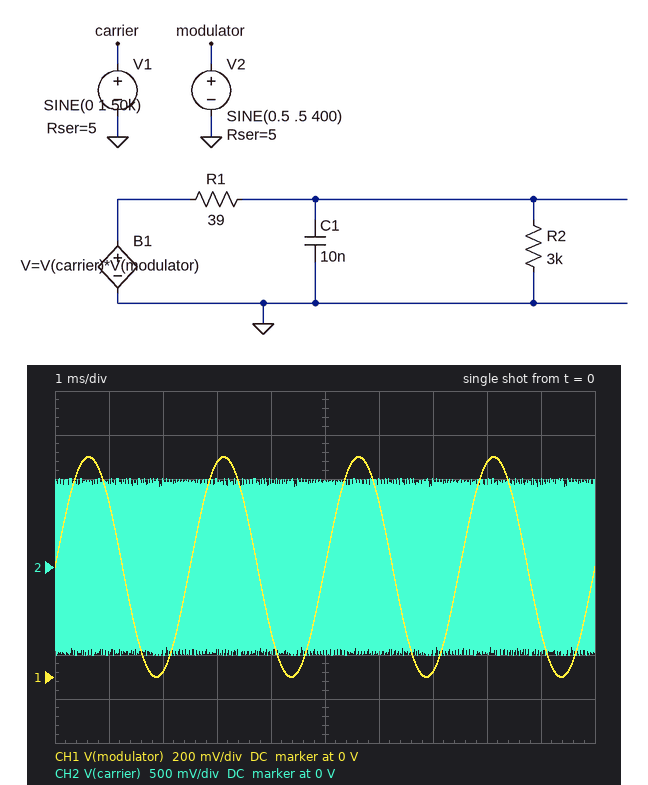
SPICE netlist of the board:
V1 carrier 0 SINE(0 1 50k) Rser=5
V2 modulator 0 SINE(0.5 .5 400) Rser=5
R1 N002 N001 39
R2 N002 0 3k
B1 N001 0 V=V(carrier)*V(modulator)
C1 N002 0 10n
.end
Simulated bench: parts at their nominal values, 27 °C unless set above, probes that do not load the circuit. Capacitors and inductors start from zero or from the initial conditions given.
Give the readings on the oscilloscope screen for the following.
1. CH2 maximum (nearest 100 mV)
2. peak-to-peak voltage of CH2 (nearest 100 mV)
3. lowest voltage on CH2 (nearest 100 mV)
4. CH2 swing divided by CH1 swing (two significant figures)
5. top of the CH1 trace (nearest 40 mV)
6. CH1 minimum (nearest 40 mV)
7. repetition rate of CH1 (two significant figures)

1.0 V
2.0 V
-1.0 V
2.0
1.00 V
0 V
400 Hz
